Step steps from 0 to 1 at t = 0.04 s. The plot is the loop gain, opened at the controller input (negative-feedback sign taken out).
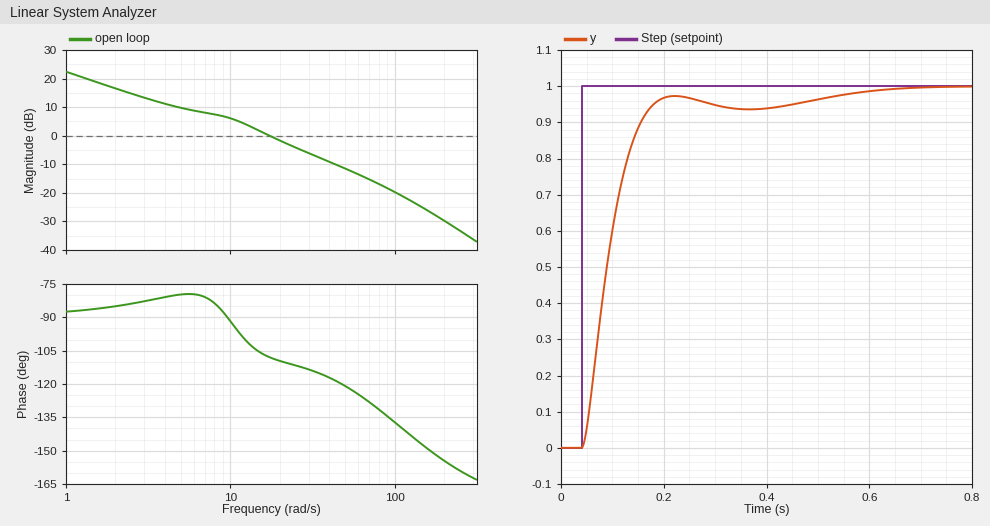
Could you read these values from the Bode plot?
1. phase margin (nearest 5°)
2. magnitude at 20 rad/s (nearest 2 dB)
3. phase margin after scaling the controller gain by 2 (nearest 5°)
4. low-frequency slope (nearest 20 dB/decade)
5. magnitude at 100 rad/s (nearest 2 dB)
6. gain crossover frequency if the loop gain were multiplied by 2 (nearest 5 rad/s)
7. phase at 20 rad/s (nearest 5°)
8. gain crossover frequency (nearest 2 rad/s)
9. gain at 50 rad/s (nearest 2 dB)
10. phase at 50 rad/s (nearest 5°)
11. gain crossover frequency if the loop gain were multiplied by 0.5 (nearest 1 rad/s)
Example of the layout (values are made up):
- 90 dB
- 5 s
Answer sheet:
- 70°
- -2 dB
- 65°
- -20 dB/decade
- -20 dB
- 30 rad/s
- -110°
- 18 rad/s
- -12 dB
- -120°
- 10 rad/s
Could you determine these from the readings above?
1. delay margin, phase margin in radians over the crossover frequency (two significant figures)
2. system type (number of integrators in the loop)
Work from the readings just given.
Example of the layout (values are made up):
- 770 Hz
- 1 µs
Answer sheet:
- 0.068 s
- 1
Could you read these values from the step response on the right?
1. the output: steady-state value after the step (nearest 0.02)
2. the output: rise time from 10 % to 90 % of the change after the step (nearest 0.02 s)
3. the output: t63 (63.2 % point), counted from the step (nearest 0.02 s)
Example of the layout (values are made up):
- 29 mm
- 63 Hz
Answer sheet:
- 1.00
- 0.10 s
- 0.06 s
